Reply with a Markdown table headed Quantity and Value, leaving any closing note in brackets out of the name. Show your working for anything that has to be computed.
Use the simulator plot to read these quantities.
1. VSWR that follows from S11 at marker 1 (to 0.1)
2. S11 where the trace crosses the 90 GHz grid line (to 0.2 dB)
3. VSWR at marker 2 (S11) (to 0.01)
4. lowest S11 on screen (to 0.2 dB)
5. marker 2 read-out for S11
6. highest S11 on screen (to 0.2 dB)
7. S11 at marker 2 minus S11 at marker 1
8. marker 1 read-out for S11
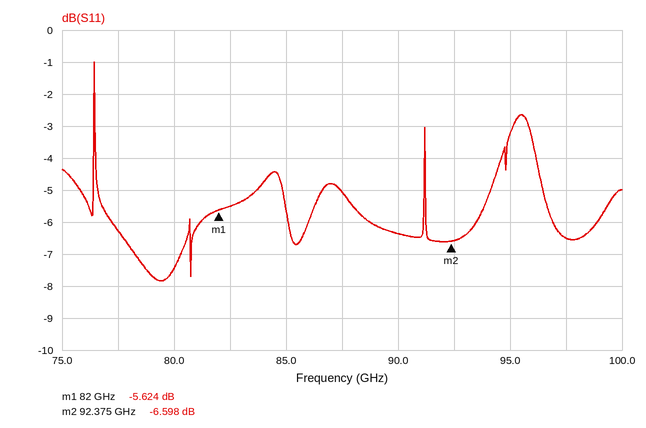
| Quantity | Value |
|---|---|
| VSWR that follows from S11 at marker 1 | (1 + 0.5234)/(1 − 0.5234) ≈ 3.2 |
| S11 where the trace crosses the 90 GHz grid line | -6.4 dB |
| VSWR at marker 2 (S11) | (1 + 0.4678)/(1 − 0.4678) ≈ 2.76 |
| lowest S11 on screen | -7.8 dB |
| marker 2 read-out for S11 | -6.598 dB |
| highest S11 on screen | -1.0 dB |
| S11 at marker 2 minus S11 at marker 1 | -6.598 − (-5.624) = -0.974 dB |
| marker 1 read-out for S11 | -5.624 dB |
